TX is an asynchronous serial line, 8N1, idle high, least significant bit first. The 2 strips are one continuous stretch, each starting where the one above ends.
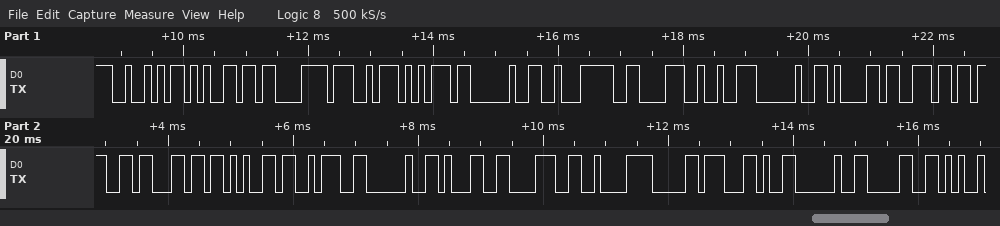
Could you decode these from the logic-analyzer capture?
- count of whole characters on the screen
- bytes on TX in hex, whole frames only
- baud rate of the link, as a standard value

24
52 65 C3 A7 75 20 E2 86 92 20 61 6E 67 6C 65 3A 20 31 38 C2 B0 2C 20 30
9600 baud
